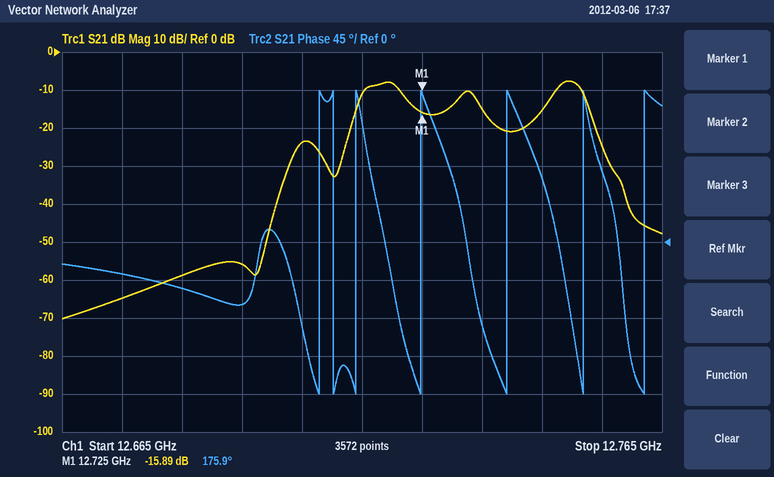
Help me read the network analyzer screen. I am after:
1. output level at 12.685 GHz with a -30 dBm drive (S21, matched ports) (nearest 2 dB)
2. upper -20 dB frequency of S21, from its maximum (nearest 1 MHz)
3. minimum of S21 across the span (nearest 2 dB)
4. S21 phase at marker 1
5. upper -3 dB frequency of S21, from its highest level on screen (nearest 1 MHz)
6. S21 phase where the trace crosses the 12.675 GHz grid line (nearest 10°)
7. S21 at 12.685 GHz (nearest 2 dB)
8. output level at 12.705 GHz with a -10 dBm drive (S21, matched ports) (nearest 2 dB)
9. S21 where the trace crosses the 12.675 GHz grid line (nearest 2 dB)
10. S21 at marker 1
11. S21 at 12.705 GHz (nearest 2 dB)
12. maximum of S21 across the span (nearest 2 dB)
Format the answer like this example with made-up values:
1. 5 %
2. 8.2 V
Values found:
1. -88 dBm
2. 12.756 GHz
3. -70 dB
4. 175.9°
5. 12.752 GHz
6. -40°
7. -58 dB
8. -34 dBm
9. -64 dB
10. -15.89 dB
11. -24 dB
12. -8 dB
